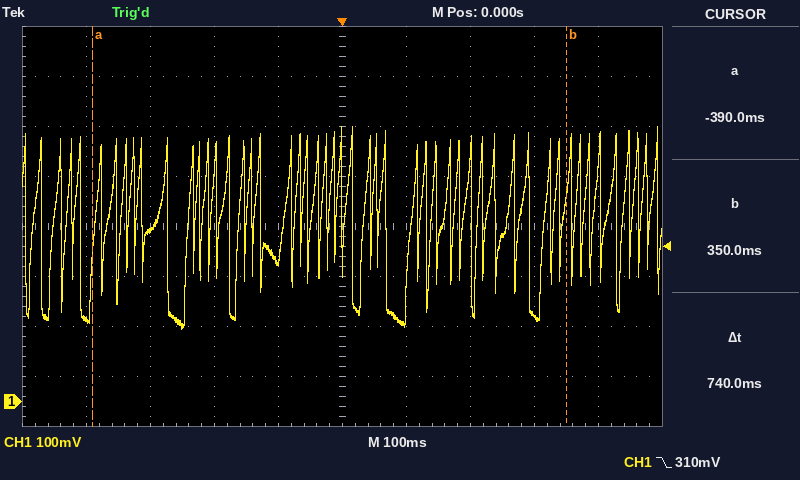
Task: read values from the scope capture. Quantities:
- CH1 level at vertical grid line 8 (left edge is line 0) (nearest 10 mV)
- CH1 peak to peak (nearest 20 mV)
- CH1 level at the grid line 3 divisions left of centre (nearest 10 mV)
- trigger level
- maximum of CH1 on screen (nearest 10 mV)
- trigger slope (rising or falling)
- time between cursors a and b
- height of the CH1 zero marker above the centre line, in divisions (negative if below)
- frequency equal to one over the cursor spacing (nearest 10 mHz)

170 mV
400 mV
340 mV
310 mV
550 mV
falling
740 ms
-3.5 div
1.35 Hz
